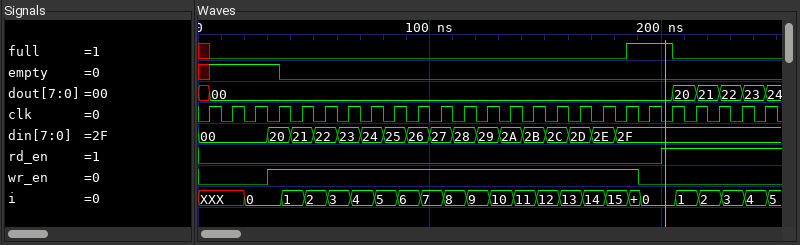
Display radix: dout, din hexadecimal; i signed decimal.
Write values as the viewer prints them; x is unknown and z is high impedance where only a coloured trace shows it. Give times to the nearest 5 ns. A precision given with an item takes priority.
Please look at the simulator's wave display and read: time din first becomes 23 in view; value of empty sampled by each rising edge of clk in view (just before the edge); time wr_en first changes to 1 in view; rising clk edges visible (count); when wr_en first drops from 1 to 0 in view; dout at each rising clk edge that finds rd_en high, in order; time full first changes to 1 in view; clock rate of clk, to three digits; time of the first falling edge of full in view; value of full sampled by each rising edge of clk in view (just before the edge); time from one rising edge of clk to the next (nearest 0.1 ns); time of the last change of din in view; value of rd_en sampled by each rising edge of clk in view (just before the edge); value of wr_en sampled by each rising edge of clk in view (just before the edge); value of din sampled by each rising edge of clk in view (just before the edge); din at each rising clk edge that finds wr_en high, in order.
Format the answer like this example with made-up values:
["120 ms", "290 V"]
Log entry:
["60 ns", "x 1 1 1 0 0 0 0 0 0 0 0 0 0 0 0 0 0 0 0 0 0 0 0 0", "30 ns", "25", "190 ns", "00, 20, 21, 22, 23", "185 ns", "100 MHz", "205 ns", "x 0 0 0 0 0 0 0 0 0 0 0 0 0 0 0 0 0 0 1 1 0 0 0 0", "10 ns", "180 ns", "0 0 0 0 0 0 0 0 0 0 0 0 0 0 0 0 0 0 0 0 1 1 1 1 1", "0 0 0 1 1 1 1 1 1 1 1 1 1 1 1 1 1 1 1 0 0 0 0 0 0", "00, 00, 00, 20, 21, 22, 23, 24, 25, 26, 27, 28, 29, 2A, 2B, 2C, 2D, 2E, 2F, 2F, 2F, 2F, 2F, 2F, 2F", "20, 21, 22, 23, 24, 25, 26, 27, 28, 29, 2A, 2B, 2C, 2D, 2E, 2F"]
